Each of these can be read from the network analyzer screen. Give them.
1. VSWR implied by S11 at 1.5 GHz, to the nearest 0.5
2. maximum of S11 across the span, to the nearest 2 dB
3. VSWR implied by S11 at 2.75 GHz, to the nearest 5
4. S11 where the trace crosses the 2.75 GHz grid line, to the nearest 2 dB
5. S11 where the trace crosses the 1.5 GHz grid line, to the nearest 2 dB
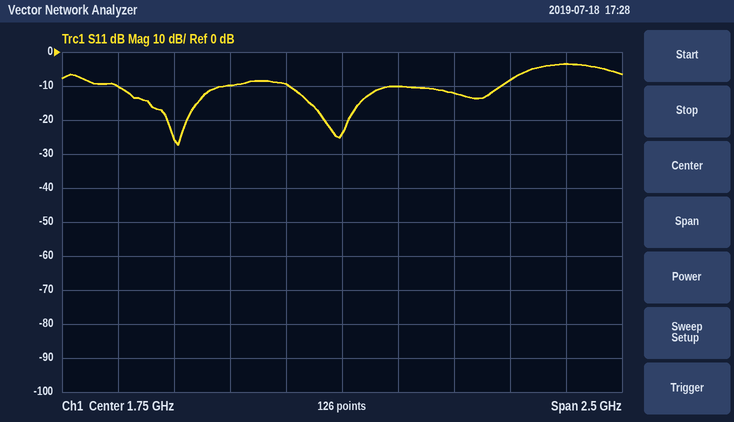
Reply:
2.0
-4 dB
5
-4 dB
-10 dB
